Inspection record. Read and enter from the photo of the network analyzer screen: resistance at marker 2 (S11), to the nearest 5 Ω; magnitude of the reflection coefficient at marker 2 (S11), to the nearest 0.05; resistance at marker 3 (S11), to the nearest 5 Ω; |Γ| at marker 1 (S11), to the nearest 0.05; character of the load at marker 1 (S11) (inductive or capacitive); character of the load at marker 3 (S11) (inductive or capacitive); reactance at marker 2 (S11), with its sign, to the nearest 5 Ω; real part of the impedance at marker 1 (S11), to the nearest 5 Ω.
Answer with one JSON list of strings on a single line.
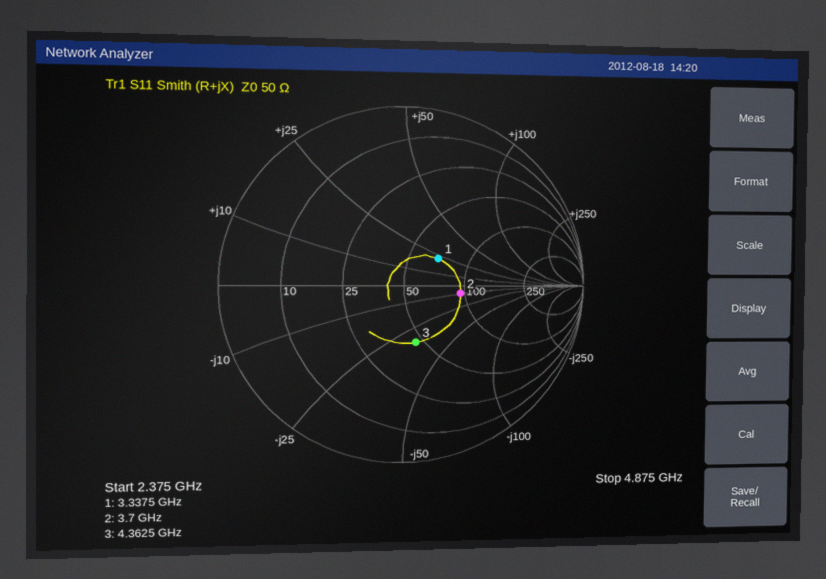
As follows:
["95 Ω", "0.30", "45 Ω", "0.25", "inductive", "capacitive", "-10 Ω", "70 Ω"]
